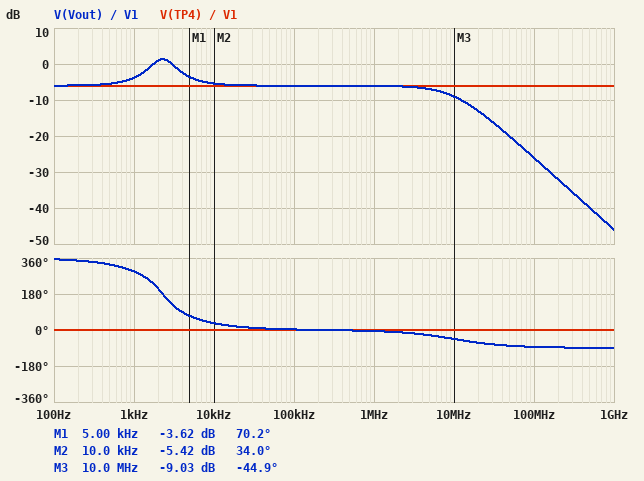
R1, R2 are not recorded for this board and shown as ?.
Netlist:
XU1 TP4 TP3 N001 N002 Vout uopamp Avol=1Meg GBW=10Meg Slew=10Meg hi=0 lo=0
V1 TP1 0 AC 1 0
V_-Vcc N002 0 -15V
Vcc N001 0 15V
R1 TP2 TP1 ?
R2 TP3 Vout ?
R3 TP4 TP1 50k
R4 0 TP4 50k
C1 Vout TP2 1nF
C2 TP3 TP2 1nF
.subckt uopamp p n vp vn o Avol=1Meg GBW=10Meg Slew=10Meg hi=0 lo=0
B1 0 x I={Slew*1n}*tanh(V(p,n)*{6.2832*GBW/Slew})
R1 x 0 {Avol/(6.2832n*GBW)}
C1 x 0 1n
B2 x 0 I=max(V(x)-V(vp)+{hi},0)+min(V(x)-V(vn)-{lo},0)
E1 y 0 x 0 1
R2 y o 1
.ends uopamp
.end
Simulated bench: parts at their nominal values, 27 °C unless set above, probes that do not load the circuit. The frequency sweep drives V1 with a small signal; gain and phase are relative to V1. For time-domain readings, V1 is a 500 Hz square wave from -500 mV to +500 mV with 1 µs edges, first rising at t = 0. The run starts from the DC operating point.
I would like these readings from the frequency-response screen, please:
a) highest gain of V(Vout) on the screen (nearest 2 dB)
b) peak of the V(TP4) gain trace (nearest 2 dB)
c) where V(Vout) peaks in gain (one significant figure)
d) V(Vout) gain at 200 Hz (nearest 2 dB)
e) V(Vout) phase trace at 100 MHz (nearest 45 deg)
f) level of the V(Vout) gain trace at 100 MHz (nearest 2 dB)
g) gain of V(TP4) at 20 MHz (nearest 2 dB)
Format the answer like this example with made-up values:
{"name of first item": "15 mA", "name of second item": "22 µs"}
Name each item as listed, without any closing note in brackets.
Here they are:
{"highest gain of V(Vout) on the screen": "2 dB", "peak of the V(TP4) gain trace": "-6 dB", "where V(Vout) peaks in gain": "2 kHz", "V(Vout) gain at 200 Hz": "-6 dB", "V(Vout) phase trace at 100 MHz": "-90 deg", "level of the V(Vout) gain trace at 100 MHz": "-26 dB", "gain of V(TP4) at 20 MHz": "-6 dB"}
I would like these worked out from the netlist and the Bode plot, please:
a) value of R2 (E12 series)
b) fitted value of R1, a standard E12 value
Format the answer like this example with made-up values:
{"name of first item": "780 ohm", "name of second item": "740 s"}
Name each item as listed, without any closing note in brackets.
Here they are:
{"value of R2": "180 kΩ", "fitted value of R1, a standard E12 value": "27 kΩ"}
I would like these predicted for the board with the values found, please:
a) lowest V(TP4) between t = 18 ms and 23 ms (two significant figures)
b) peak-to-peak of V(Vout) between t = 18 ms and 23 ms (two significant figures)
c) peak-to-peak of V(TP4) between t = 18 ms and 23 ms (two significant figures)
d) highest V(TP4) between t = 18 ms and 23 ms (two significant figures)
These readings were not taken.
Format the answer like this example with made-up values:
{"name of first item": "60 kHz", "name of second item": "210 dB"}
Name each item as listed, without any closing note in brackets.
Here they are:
{"lowest V(TP4) between t = 18 ms and 23 ms": "-250 mV", "peak-to-peak of V(Vout) between t = 18 ms and 23 ms": "1.1 V", "peak-to-peak of V(TP4) between t = 18 ms and 23 ms": "500 mV", "highest V(TP4) between t = 18 ms and 23 ms": "250 mV"}
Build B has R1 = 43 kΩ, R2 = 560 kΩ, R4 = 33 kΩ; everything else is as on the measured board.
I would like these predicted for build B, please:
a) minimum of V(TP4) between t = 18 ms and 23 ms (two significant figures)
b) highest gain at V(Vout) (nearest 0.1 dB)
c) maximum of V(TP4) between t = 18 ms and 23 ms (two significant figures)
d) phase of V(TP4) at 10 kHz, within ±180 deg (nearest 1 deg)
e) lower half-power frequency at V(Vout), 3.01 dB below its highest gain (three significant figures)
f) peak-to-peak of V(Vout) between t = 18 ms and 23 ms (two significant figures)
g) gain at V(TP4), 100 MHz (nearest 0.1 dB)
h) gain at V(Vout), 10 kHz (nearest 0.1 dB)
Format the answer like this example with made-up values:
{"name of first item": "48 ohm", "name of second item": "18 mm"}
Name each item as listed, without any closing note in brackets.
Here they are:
{"minimum of V(TP4) between t = 18 ms and 23 ms": "-200 mV", "highest gain at V(Vout)": "10.9 dB", "maximum of V(TP4) between t = 18 ms and 23 ms": "200 mV", "phase of V(TP4) at 10 kHz, within ±180 deg": "0 deg", "lower half-power frequency at V(Vout), 3.01 dB below its highest gain": "777 Hz", "peak-to-peak of V(Vout) between t = 18 ms and 23 ms": "2.2 V", "gain at V(TP4), 100 MHz": "-8.0 dB", "gain at V(Vout), 10 kHz": "-7.0 dB"}
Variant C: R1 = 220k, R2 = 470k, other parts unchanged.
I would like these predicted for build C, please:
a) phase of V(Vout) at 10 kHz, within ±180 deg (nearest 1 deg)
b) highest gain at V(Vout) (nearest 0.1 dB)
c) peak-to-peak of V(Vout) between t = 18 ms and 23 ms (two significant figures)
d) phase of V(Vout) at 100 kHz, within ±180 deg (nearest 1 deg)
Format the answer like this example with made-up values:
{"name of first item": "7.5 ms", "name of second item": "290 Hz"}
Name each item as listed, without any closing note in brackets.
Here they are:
{"phase of V(Vout) at 10 kHz, within ±180 deg": "4 deg", "highest gain at V(Vout)": "-6.0 dB", "peak-to-peak of V(Vout) between t = 18 ms and 23 ms": "710 mV", "phase of V(Vout) at 100 kHz, within ±180 deg": "0 deg"}
